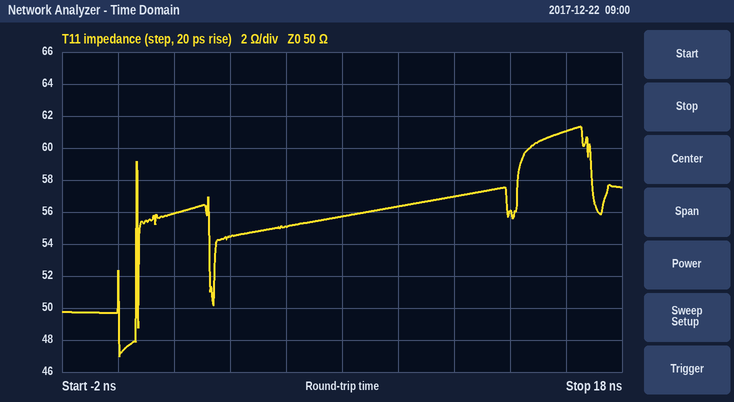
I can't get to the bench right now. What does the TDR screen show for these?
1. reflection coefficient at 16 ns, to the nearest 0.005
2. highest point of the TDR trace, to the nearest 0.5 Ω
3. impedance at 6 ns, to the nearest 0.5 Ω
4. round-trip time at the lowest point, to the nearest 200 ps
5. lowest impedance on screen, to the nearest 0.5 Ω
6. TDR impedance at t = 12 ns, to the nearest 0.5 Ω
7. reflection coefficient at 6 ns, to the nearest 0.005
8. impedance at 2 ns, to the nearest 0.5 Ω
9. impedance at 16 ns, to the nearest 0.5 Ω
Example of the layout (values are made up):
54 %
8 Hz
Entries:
+0.100
61.5 Ω
55.0 Ω
0.0 ns
47.0 Ω
57.0 Ω
+0.050
56.0 Ω
61.0 Ω
